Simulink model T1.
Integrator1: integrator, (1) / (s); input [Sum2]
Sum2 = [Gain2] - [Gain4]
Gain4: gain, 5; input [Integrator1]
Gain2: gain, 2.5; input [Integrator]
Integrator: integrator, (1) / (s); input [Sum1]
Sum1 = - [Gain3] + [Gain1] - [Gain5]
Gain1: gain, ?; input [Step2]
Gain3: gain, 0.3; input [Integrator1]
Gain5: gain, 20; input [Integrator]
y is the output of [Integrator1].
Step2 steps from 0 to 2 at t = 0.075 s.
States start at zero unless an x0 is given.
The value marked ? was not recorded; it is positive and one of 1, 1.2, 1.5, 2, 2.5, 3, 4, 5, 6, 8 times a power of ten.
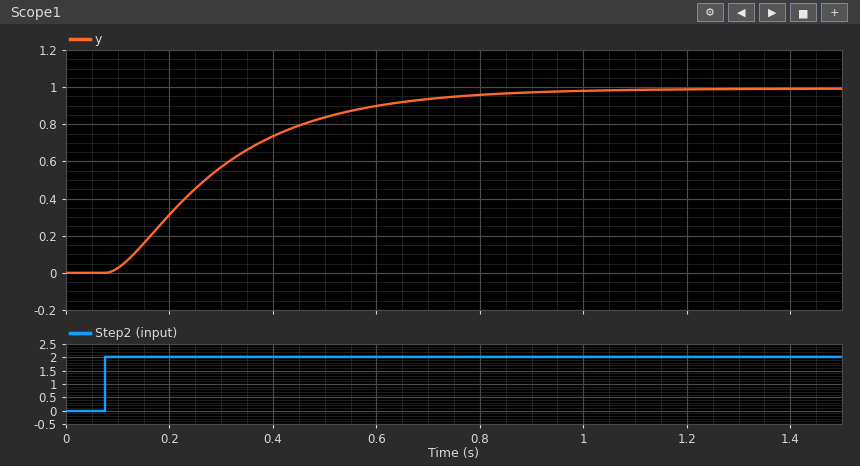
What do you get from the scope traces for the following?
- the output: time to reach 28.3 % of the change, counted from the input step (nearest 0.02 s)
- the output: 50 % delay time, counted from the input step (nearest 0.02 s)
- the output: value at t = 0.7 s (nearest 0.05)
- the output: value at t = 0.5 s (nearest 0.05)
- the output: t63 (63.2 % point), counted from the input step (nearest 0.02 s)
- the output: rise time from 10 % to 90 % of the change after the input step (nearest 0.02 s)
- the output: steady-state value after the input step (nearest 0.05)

0.12 s
0.20 s
0.95
0.85
0.26 s
0.46 s
1.00
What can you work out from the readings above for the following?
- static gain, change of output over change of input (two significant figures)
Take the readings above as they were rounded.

0.50
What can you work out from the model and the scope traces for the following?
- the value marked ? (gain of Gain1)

20
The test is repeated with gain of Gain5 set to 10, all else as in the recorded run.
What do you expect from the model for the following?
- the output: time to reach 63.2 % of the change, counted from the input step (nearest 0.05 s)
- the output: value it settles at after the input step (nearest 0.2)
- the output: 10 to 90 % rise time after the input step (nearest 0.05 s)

0.30 s
2.0
0.50 s
